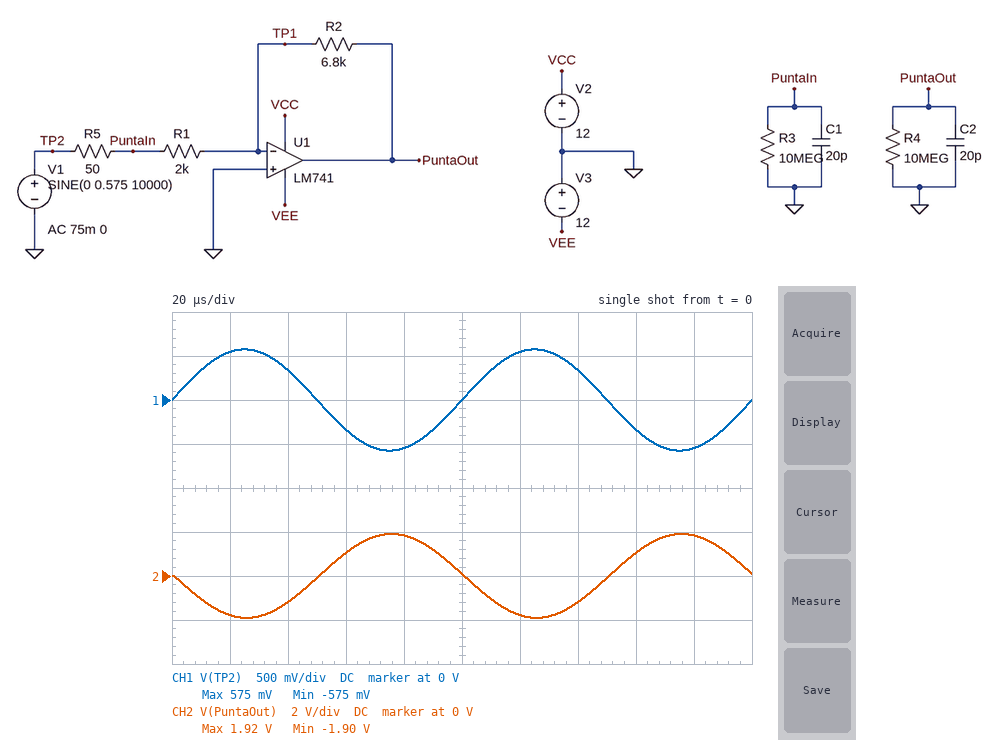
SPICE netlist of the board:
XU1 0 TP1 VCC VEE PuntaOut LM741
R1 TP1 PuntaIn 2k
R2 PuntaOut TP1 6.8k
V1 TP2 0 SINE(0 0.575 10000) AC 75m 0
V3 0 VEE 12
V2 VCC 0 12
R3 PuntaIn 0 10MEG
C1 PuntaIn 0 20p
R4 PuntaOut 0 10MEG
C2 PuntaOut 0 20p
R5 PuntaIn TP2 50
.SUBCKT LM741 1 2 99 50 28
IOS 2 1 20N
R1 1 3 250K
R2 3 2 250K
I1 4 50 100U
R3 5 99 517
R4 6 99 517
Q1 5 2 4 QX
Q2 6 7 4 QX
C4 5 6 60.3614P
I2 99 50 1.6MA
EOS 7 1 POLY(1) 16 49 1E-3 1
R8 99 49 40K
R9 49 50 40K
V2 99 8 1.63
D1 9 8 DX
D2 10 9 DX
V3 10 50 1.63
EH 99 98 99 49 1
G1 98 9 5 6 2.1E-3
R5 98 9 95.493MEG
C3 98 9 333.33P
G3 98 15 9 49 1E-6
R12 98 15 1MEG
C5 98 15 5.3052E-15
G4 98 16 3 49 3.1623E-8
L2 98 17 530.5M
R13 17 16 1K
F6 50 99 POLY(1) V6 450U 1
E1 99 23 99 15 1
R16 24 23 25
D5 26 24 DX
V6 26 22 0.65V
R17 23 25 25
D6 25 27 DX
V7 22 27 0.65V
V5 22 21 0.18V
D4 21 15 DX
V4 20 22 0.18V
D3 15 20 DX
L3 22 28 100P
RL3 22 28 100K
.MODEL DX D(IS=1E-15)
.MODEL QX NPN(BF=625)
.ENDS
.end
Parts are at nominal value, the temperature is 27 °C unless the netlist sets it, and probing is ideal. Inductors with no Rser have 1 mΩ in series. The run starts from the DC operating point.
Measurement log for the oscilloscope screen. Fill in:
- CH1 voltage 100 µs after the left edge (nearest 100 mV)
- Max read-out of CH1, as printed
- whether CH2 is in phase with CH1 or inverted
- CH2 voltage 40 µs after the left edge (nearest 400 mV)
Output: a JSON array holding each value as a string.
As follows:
["0 V", "575 mV", "inverted", "-1.2 V"]
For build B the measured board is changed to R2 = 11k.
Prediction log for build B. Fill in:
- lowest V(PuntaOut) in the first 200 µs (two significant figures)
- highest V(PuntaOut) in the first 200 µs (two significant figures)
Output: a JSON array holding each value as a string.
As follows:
["-3.1 V", "3.1 V"]
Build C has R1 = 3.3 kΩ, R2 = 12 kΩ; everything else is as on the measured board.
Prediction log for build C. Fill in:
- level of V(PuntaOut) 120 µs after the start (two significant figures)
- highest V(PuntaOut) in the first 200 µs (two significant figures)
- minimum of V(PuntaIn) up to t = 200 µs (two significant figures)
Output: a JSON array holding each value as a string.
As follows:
["-1.9 V", "2.1 V", "-570 mV"]
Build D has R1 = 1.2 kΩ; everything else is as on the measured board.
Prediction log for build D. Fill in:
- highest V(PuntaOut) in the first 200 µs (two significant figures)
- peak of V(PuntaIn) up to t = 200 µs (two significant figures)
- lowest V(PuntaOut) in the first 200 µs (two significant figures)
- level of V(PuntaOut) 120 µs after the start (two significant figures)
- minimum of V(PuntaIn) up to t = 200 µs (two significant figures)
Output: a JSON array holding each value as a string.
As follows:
["3.1 V", "550 mV", "-3.1 V", "-2.9 V", "-550 mV"]
